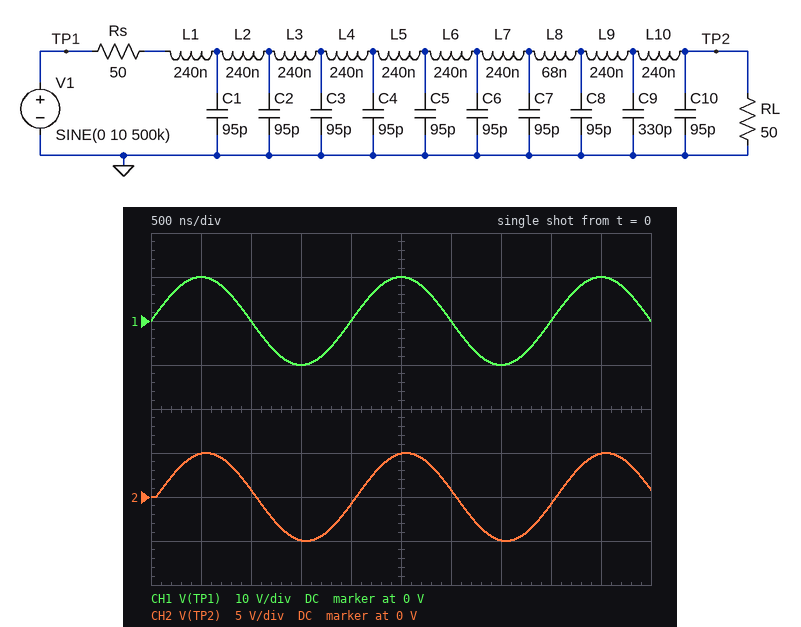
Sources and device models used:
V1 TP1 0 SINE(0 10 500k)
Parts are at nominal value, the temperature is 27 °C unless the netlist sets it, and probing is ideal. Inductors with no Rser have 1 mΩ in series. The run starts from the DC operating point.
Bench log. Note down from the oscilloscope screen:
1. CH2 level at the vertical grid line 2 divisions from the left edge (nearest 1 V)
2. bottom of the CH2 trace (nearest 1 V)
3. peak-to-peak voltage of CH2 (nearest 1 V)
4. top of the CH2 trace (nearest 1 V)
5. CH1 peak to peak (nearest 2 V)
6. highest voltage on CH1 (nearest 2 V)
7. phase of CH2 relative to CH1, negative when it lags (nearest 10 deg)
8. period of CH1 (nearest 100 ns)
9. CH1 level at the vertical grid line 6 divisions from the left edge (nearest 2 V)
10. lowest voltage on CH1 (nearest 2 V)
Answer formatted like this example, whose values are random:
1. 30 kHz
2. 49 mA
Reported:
1. 1 V
2. -5 V
3. 10 V
4. 5 V
5. 20 V
6. 10 V
7. -10 deg
8. 2.0 µs
9. 0 V
10. -10 V
